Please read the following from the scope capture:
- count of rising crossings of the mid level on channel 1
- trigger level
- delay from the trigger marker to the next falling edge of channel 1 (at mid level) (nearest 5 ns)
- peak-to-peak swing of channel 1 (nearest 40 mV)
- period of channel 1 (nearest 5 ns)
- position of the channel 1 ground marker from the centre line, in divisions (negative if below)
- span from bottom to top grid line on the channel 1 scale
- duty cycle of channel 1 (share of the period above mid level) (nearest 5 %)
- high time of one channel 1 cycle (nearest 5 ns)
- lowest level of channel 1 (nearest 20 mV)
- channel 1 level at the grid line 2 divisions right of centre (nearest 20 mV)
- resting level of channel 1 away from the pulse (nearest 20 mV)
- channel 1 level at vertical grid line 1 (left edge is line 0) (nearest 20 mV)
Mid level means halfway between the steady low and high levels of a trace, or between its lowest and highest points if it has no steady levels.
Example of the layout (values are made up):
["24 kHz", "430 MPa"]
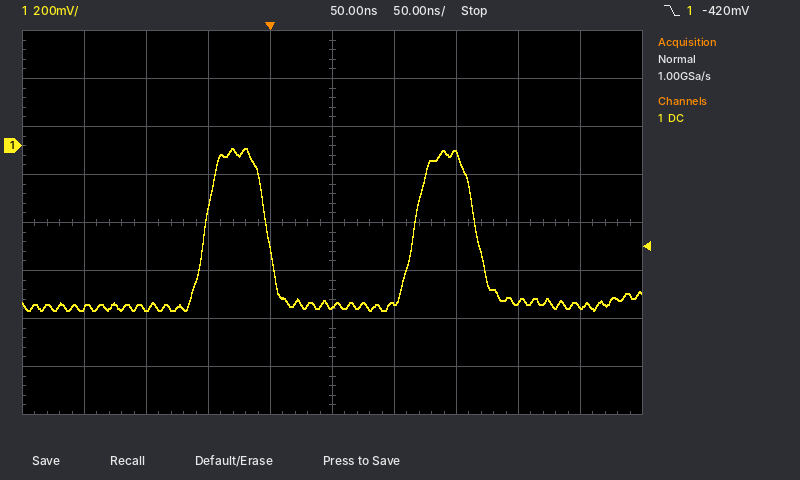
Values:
["2", "-420 mV", "165 ns", "680 mV", "170 ns", "+1.6 div", "1.6 V", "30 %", "50 ns", "-680 mV", "-40 mV", "-660 mV", "-680 mV"]
